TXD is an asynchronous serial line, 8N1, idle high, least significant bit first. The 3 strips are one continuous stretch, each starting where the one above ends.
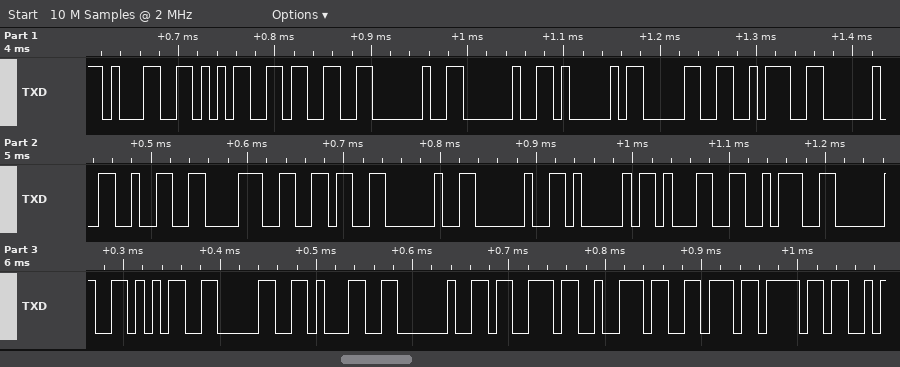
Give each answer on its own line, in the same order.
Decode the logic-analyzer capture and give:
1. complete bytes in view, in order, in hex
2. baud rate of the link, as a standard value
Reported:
31 35 33 20 20 41 30 3A 20 32 38 36 20 20 41 31 3A 20 35 30 31 20 73 72 76 6F
115200 baud
